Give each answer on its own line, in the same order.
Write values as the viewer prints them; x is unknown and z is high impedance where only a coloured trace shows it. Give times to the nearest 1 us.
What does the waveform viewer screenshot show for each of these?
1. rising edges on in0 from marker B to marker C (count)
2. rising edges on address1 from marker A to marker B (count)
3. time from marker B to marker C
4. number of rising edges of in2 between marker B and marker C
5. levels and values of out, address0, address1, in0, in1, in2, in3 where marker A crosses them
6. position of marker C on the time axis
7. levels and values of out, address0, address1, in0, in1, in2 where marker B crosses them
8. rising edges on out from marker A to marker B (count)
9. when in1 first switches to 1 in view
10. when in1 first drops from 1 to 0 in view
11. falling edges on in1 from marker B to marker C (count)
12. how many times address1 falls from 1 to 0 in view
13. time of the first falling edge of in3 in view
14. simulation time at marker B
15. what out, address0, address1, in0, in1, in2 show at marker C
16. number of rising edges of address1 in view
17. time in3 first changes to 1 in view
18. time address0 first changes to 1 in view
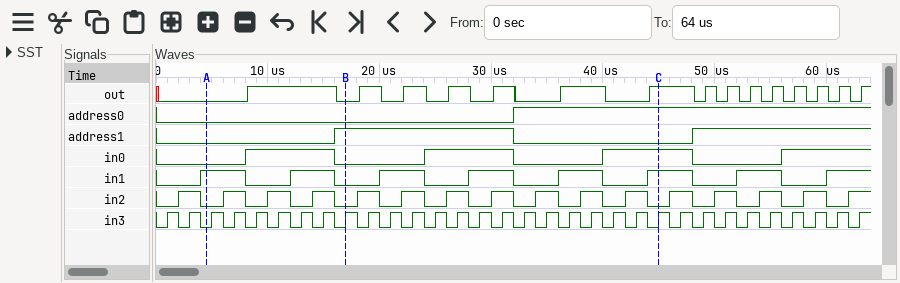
2
1
28 us
7
out=0, address0=0, address1=0, in0=0, in1=1, in2=0, in3=0
45 us
out=0, address0=0, address1=1, in0=0, in1=0, in2=0
1
4 us
8 us
3
1
2 us
17 us
out=1, address0=1, address1=0, in0=1, in1=1, in2=0
2
1 us
32 us
